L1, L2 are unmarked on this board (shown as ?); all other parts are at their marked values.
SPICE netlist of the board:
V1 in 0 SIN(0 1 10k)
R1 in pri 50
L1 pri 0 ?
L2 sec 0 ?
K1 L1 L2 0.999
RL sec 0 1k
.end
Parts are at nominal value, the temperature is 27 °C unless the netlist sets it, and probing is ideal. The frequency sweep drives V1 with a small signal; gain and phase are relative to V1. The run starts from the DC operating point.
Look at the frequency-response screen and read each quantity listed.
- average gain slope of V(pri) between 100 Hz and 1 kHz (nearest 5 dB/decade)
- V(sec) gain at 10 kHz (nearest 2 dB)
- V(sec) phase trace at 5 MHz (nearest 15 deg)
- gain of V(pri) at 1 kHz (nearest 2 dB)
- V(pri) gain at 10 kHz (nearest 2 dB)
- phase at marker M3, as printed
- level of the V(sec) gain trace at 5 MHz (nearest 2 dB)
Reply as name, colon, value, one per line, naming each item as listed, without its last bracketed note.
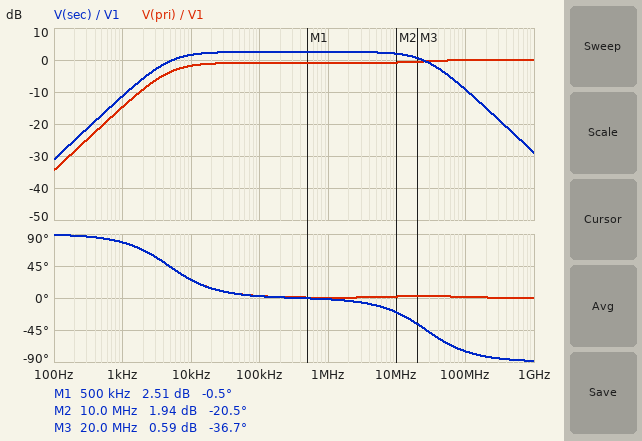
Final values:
average gain slope of V(pri) between 100 Hz and 1 kHz: 20 dB/decade
V(sec) gain at 10 kHz: 2 dB
V(sec) phase trace at 5 MHz: -15 deg
gain of V(pri) at 1 kHz: -14 dB
V(pri) gain at 10 kHz: -2 dB
phase at marker M3, as printed: -36.7 deg
level of the V(sec) gain trace at 5 MHz: 2 dB
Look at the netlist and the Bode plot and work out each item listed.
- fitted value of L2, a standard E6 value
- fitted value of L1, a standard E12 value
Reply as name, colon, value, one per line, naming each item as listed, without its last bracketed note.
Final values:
fitted value of L2, a standard E6 value: 3.3 mH
fitted value of L1, a standard E12 value: 1.5 mH
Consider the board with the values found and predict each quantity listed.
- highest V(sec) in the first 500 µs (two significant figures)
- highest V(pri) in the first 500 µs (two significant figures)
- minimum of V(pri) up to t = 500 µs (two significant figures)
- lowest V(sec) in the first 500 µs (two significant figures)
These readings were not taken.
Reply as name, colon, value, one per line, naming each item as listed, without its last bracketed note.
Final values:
highest V(sec) in the first 500 µs: 1.2 V
highest V(pri) in the first 500 µs: 810 mV
minimum of V(pri) up to t = 500 µs: -860 mV
lowest V(sec) in the first 500 µs: -1.3 V
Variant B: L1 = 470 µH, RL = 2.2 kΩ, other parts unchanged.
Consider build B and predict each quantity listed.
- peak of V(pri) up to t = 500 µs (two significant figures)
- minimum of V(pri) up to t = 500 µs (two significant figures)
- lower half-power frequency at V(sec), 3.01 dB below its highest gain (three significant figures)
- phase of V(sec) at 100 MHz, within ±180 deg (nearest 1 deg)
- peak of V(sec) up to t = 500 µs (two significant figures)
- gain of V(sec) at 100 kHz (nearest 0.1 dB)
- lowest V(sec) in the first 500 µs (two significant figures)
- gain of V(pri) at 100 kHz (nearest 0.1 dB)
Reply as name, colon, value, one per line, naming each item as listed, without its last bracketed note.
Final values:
peak of V(pri) up to t = 500 µs: 490 mV
minimum of V(pri) up to t = 500 µs: -490 mV
lower half-power frequency at V(sec), 3.01 dB below its highest gain: 14.6 kHz
phase of V(sec) at 100 MHz, within ±180 deg: -58 deg
peak of V(sec) up to t = 500 µs: 1.3 V
gain of V(sec) at 100 kHz: 7.1 dB
lowest V(sec) in the first 500 µs: -1.3 V
gain of V(pri) at 100 kHz: -1.4 dB
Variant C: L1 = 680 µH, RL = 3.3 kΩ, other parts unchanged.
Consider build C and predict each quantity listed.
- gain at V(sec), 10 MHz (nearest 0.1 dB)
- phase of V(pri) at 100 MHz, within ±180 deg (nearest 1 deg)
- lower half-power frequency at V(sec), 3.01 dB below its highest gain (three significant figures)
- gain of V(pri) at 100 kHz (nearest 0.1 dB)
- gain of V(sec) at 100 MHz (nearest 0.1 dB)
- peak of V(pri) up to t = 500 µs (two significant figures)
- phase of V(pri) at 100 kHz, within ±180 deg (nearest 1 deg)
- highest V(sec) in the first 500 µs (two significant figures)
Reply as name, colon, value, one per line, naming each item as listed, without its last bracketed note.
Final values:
gain at V(sec), 10 MHz: 6.2 dB
phase of V(pri) at 100 MHz, within ±180 deg: 2 deg
lower half-power frequency at V(sec), 3.01 dB below its highest gain: 10.9 kHz
gain of V(pri) at 100 kHz: -0.7 dB
gain of V(sec) at 100 MHz: 2.5 dB
peak of V(pri) up to t = 500 µs: 630 mV
phase of V(pri) at 100 kHz, within ±180 deg: 6 deg
highest V(sec) in the first 500 µs: 1.4 V
